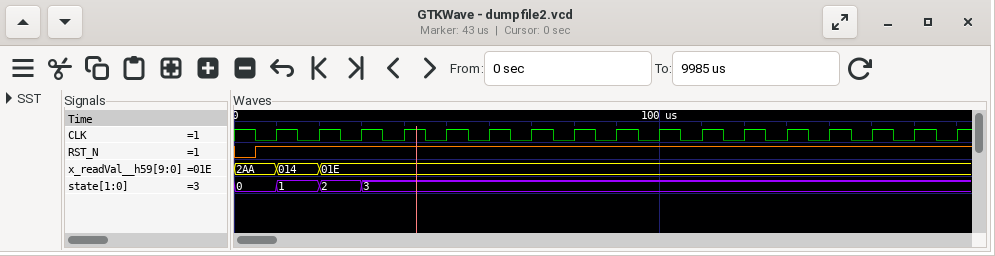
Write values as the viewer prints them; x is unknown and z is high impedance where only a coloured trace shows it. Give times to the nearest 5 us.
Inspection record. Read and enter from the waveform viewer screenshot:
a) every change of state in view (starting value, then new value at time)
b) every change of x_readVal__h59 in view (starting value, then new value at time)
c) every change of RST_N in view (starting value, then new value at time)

0, 1 at 10 us, 2 at 20 us, 3 at 30 us
2AA, 014 at 10 us, 01E at 20 us
0, 1 at 5 us
